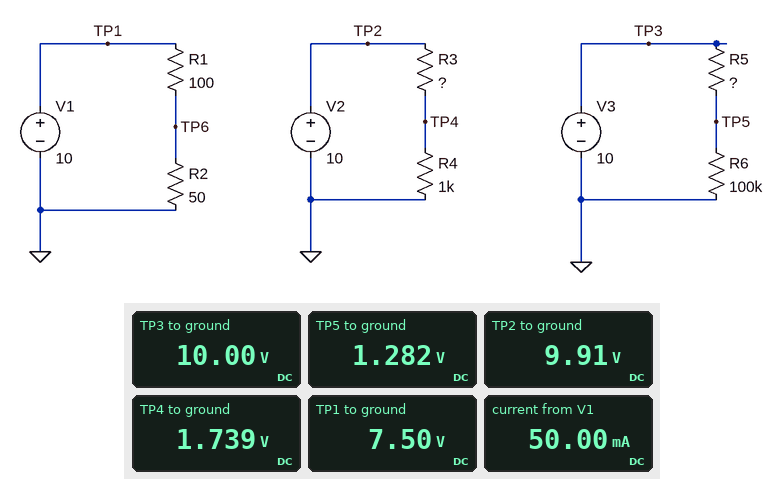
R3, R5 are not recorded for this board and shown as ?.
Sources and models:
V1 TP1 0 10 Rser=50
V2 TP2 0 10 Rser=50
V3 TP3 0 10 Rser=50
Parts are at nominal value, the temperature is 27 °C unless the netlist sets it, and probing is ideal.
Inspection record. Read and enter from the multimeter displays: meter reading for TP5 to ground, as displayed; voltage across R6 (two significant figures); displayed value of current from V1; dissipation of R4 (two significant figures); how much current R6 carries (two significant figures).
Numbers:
1.282 V
1.3 V
50.00 mA
3.0 mW
13 µA
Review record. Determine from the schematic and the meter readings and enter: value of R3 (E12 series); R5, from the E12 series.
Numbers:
4.7 kΩ
680 kΩ
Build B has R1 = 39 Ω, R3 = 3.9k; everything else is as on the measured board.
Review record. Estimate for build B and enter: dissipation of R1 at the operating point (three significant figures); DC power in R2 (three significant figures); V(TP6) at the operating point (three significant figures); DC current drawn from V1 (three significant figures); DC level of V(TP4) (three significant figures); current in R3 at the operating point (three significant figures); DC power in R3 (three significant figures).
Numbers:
202 mW
259 mW
3.60 V
71.9 mA
2.02 V
2.02 mA
15.9 mW
